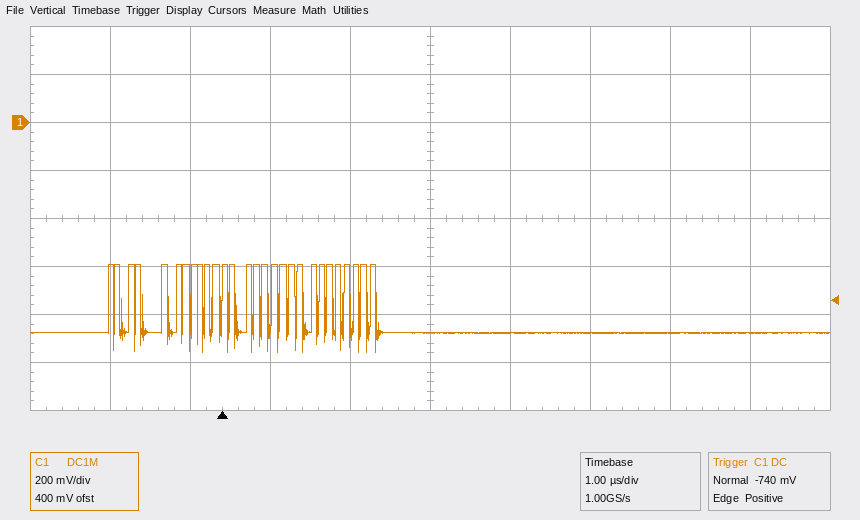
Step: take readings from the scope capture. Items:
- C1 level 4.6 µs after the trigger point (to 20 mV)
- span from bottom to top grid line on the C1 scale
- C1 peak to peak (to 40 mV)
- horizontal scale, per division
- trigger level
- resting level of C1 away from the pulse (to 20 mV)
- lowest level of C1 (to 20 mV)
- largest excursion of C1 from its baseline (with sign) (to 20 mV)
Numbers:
-880 mV
1.6 V
360 mV
1 µs
-740 mV
-880 mV
-960 mV
+280 mV
